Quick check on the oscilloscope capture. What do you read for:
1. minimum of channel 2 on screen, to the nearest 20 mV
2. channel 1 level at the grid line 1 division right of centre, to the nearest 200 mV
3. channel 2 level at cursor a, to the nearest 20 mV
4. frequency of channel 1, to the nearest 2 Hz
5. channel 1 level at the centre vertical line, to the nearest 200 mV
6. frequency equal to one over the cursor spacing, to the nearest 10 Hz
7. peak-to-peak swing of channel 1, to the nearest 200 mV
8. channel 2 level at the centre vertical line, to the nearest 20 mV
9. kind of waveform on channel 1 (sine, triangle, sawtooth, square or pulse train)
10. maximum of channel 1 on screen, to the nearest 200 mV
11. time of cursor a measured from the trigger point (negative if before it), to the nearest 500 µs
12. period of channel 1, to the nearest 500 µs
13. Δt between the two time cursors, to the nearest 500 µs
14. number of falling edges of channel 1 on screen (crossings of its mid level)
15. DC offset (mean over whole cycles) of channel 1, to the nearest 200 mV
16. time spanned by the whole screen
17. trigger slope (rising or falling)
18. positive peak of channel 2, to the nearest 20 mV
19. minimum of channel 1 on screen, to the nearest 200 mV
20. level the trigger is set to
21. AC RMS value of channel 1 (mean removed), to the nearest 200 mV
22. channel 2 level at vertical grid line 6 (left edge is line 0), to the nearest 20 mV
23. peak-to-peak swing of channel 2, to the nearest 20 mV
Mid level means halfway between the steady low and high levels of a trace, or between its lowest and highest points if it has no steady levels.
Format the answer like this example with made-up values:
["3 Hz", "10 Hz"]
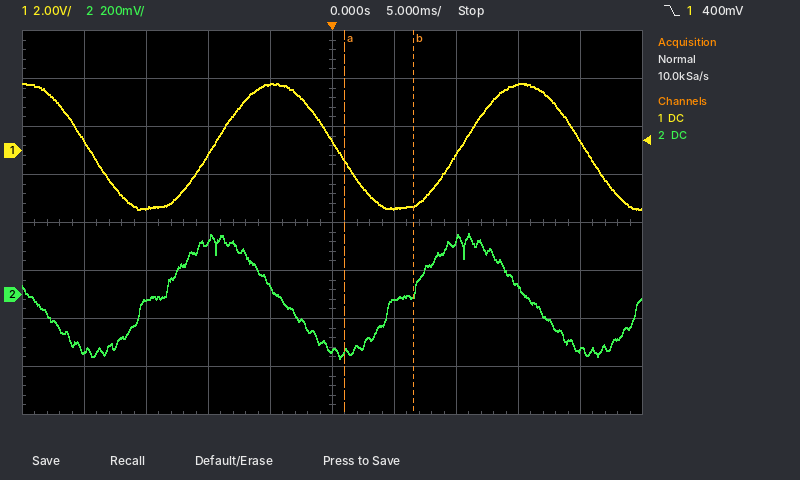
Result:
["-260 mV", "-2.4 V", "-240 mV", "50 Hz", "400 mV", "180 Hz", "5.2 V", "-240 mV", "sine", "2.8 V", "+1.0 ms", "20.0 ms", "5.5 ms", "3", "200 mV", "50 ms", "falling", "260 mV", "-2.4 V", "400 mV", "1.8 V", "-20 mV", "520 mV"]
